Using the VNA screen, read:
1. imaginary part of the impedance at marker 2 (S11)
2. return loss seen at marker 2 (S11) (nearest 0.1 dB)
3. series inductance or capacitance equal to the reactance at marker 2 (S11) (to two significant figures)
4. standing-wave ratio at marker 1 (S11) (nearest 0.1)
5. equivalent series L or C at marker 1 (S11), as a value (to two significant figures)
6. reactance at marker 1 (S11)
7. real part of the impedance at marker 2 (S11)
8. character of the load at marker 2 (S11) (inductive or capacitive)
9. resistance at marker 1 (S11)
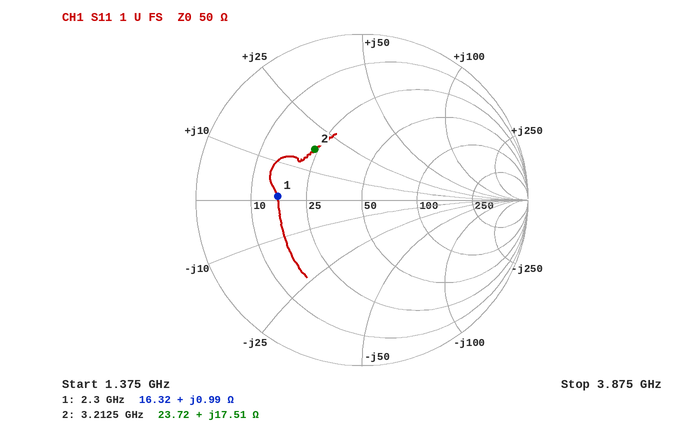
+17.51 Ω
7.6 dB
870 pH
3.1
69 pH
+0.99 Ω
23.72 Ω
inductive
16.32 Ω
